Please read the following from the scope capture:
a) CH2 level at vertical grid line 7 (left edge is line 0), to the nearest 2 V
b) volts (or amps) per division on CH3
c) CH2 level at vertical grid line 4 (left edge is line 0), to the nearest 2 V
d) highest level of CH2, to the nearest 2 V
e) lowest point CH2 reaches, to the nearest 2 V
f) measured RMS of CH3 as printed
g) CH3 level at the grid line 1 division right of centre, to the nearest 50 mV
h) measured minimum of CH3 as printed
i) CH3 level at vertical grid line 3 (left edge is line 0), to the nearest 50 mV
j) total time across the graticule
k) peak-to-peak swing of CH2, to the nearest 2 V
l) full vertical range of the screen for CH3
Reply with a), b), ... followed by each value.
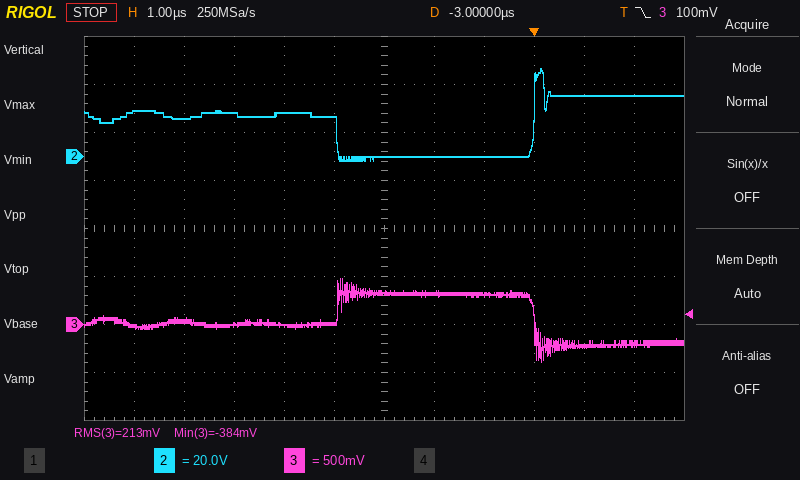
a) 0 V
b) 500 mV
c) 18 V
d) 36 V
e) -2 V
f) 213 mV
g) 350 mV
h) -384 mV
i) 0 mV
j) 12 µs
k) 38 V
l) 4 V
